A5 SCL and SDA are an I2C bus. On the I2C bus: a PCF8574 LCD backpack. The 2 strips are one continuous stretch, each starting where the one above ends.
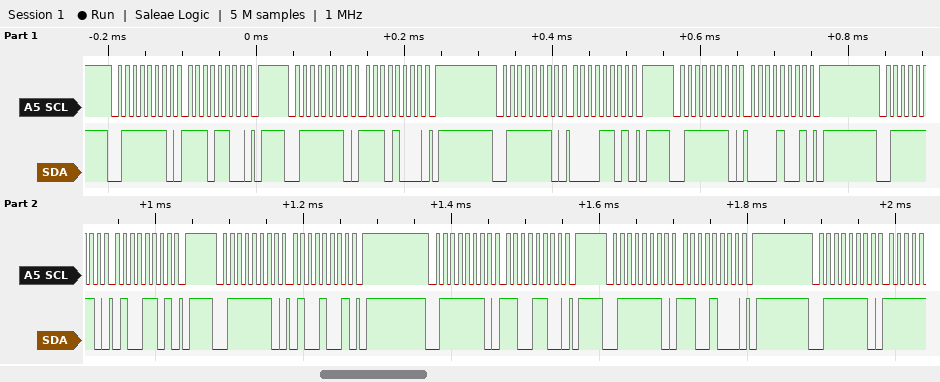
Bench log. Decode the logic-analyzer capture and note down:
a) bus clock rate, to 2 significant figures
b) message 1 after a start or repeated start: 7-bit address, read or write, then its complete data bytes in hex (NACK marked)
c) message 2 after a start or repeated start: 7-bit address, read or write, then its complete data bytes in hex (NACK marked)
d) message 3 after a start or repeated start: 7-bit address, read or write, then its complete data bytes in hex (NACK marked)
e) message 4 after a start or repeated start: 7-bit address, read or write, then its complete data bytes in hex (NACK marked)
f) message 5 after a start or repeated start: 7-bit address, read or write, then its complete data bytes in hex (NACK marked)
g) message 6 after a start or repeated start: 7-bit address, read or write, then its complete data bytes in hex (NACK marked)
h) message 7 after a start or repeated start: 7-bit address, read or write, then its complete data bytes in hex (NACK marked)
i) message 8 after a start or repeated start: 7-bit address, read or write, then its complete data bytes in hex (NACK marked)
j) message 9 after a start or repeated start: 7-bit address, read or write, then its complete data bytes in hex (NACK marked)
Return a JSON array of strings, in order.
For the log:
["100 kHz", "0x3F write: EC", "0x3F write: E8", "0x3F write: 0D", "0x3F write: 09", "0x3F write: 4D", "0x3F write: 49", "0x3F write: CC", "0x3F write: C8", "0x3F write"]
